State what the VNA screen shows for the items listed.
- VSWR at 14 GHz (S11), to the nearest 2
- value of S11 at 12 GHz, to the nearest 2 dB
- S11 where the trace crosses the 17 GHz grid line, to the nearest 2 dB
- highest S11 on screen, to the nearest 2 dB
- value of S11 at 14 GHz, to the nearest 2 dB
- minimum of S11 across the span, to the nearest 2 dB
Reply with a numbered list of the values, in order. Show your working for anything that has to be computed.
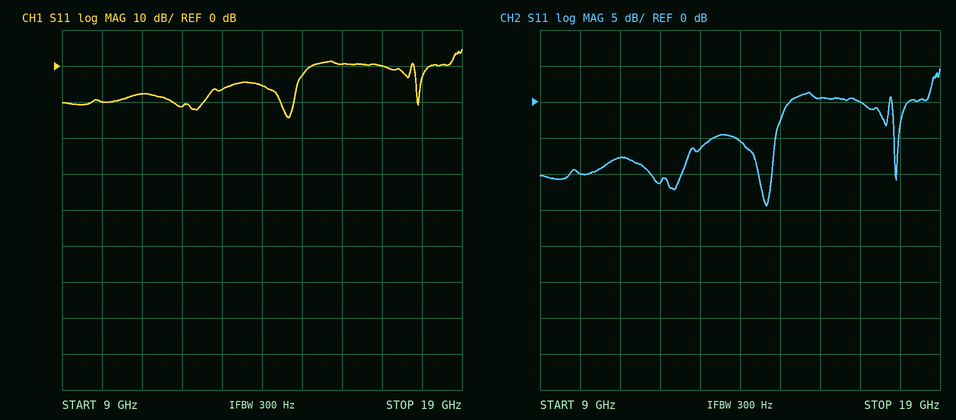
1. |Γ| = 10^(-6/20) = 0.5012; VSWR = (1 + 0.5012)/(1 − 0.5012) ≈ 3.01, so 4 to the nearest 2
2. -12 dB
3. 0 dB
4. 4 dB
5. -6 dB
6. -14 dB
